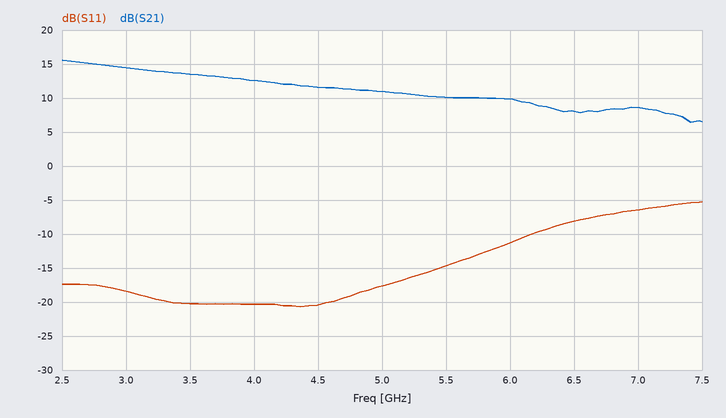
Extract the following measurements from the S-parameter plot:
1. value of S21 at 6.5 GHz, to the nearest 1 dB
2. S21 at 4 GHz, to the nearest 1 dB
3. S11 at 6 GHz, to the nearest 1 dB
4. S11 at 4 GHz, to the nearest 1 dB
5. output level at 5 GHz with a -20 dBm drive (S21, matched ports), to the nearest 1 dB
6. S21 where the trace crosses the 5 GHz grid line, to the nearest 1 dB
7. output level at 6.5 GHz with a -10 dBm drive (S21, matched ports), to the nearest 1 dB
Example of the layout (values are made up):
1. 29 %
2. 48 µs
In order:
1. 8 dB
2. 13 dB
3. -11 dB
4. -20 dB
5. -9 dBm
6. 11 dB
7. -2 dBm
